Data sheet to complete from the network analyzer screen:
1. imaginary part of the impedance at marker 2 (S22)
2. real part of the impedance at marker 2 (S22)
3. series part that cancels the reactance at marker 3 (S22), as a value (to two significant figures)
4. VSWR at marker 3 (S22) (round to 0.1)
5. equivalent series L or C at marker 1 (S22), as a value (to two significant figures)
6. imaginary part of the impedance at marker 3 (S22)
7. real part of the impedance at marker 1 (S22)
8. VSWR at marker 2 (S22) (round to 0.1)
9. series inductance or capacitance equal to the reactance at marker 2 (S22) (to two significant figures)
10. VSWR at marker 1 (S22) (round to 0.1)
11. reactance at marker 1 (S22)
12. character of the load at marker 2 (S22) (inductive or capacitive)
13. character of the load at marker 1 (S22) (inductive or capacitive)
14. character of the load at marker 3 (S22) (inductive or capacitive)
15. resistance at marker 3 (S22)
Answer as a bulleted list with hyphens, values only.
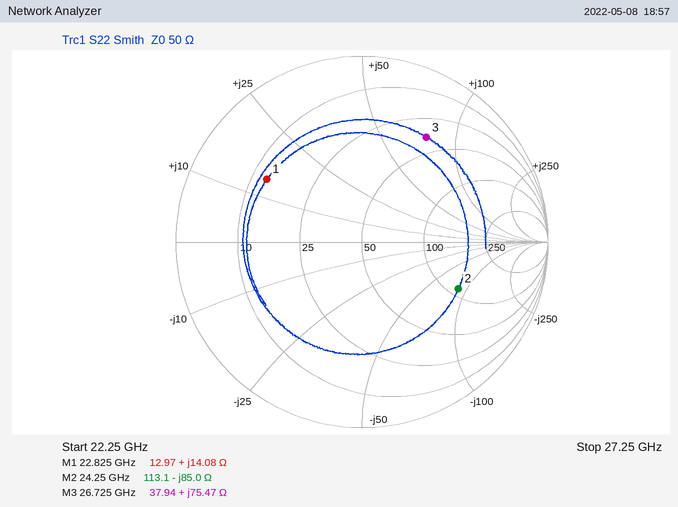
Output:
- -85.0 Ω
- 113.1 Ω
- 79 fF
- 4.9
- 98 pH
- +75.47 Ω
- 12.97 Ω
- 3.7
- 77 fF
- 4.2
- +14.08 Ω
- capacitive
- inductive
- inductive
- 37.94 Ω
